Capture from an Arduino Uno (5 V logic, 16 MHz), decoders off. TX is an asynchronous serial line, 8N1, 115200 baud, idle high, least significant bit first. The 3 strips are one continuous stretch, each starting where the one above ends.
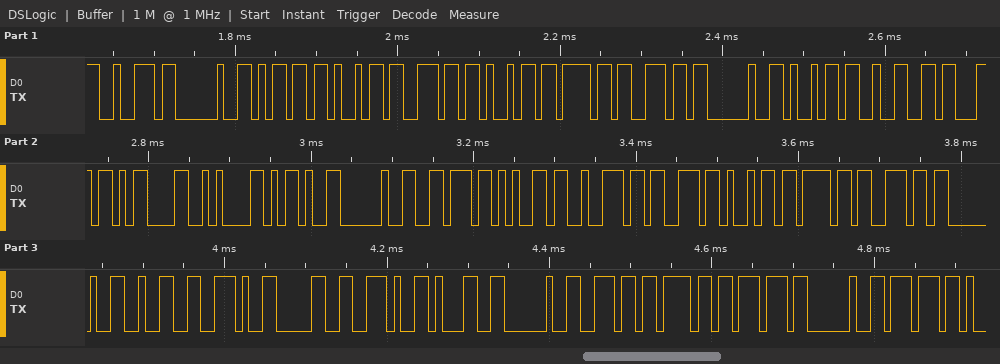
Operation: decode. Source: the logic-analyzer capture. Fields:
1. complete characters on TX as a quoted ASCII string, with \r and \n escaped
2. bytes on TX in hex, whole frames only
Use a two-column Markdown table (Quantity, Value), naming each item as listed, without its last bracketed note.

| Quantity | Value |
|---|---|
| complete characters on TX as a quoted ASCII string, with \r and \n escaped | "r minion i2c\r\n- version 2.0.1 now w" |
| bytes on TX in hex, whole frames only | 72 20 6D 69 6E 69 6F 6E 20 69 32 63 0D 0A 2D 20 76 65 72 73 69 6F 6E 20 32 2E 30 2E 31 20 6E 6F 77 20 77 |
